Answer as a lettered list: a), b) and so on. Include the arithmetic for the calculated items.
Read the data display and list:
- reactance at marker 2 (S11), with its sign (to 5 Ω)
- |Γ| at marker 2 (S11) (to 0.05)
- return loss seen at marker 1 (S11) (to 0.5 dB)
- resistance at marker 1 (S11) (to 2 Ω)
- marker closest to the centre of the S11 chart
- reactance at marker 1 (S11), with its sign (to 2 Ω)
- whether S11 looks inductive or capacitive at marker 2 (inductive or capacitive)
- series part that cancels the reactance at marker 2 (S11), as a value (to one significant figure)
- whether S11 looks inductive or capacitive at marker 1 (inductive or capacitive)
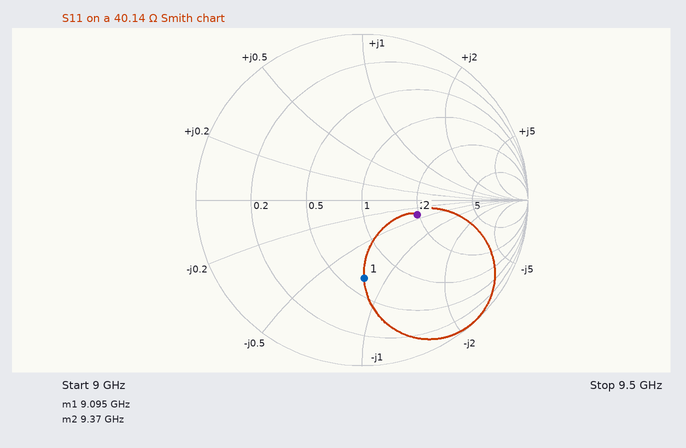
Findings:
a) -15 Ω
b) 0.35
c) 6.5 dB
d) 26 Ω
e) marker 2
f) -32 Ω
g) capacitive
h) L = 15 Ω/(2π × 9.37 GHz) ≈ 255 pH, so 300 pH to one significant figure
i) capacitive
